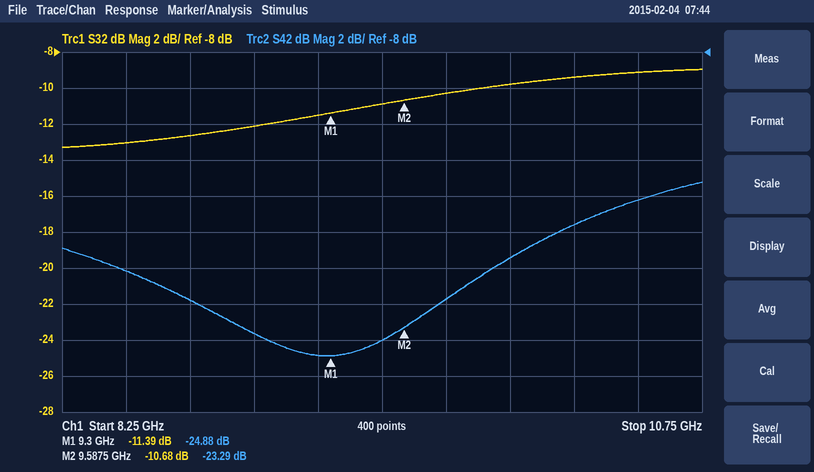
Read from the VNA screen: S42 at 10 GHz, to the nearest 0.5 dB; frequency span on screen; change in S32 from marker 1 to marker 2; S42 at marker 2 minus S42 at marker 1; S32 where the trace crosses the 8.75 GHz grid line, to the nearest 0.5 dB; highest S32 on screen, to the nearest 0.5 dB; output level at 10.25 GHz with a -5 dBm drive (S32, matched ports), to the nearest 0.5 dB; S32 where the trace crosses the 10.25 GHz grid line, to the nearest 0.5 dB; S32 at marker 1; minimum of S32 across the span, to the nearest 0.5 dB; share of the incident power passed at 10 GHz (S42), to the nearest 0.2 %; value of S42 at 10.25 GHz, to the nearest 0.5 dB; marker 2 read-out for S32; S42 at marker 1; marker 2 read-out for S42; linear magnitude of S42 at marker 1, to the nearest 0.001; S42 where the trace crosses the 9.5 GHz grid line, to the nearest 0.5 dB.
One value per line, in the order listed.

-19.5 dB
2.5 GHz
0.71 dB
1.59 dB
-12.5 dB
-9.0 dB
-14.5 dBm
-9.5 dB
-11.39 dB
-13.5 dB
1.2 %
-17.5 dB
-10.68 dB
-24.88 dB
-23.29 dB
0.057
-24.0 dB
